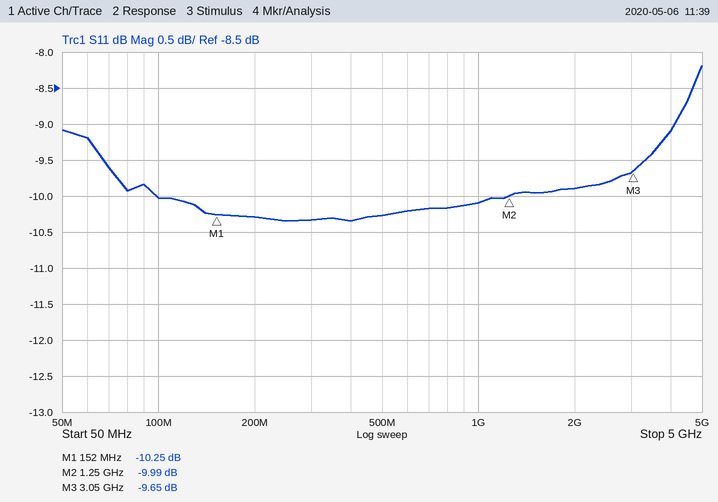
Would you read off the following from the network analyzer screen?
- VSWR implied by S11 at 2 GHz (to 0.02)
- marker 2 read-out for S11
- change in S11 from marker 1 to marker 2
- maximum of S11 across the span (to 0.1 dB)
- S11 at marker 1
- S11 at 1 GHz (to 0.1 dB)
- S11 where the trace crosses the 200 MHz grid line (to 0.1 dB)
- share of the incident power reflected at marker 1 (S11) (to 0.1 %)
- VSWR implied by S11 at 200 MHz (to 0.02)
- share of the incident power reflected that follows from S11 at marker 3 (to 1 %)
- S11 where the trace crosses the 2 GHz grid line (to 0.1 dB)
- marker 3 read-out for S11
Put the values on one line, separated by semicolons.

1.94; -9.99 dB; 0.26 dB; -8.2 dB; -10.25 dB; -10.1 dB; -10.3 dB; 9.4 %; 1.88; 11 %; -9.9 dB; -9.65 dB
